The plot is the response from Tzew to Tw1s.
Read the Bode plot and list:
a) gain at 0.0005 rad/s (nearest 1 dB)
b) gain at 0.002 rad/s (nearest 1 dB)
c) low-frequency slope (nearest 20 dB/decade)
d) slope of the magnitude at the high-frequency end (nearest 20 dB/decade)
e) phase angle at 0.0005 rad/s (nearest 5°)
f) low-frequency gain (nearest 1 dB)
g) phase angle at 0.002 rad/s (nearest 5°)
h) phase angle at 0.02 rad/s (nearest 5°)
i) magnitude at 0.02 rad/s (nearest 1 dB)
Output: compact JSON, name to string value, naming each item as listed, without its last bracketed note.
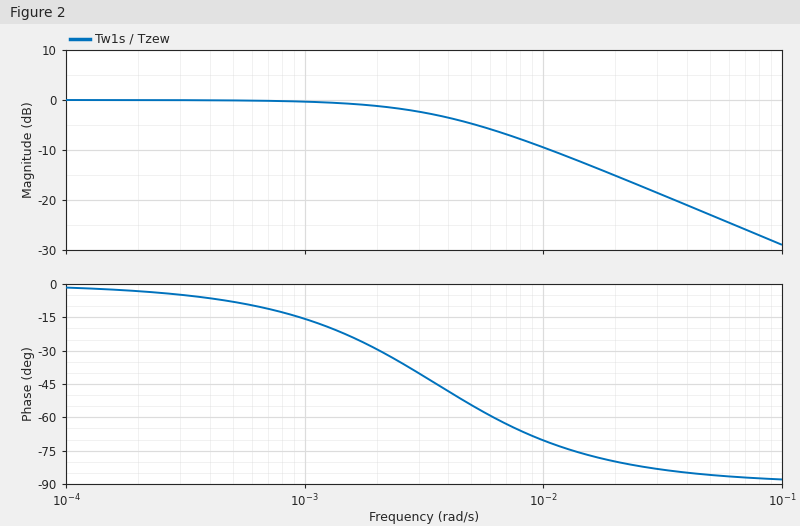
{"gain at 0.0005 rad/s": "0 dB", "gain at 0.002 rad/s": "-1 dB", "low-frequency slope": "0 dB/decade", "slope of the magnitude at the high-frequency end": "-20 dB/decade", "phase angle at 0.0005 rad/s": "-10°", "low-frequency gain": "0 dB", "phase angle at 0.002 rad/s": "-30°", "phase angle at 0.02 rad/s": "-80°", "magnitude at 0.02 rad/s": "-15 dB"}
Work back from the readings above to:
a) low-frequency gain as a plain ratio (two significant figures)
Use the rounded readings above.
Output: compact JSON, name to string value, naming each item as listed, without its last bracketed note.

{"low-frequency gain as a plain ratio": "1.0"}
